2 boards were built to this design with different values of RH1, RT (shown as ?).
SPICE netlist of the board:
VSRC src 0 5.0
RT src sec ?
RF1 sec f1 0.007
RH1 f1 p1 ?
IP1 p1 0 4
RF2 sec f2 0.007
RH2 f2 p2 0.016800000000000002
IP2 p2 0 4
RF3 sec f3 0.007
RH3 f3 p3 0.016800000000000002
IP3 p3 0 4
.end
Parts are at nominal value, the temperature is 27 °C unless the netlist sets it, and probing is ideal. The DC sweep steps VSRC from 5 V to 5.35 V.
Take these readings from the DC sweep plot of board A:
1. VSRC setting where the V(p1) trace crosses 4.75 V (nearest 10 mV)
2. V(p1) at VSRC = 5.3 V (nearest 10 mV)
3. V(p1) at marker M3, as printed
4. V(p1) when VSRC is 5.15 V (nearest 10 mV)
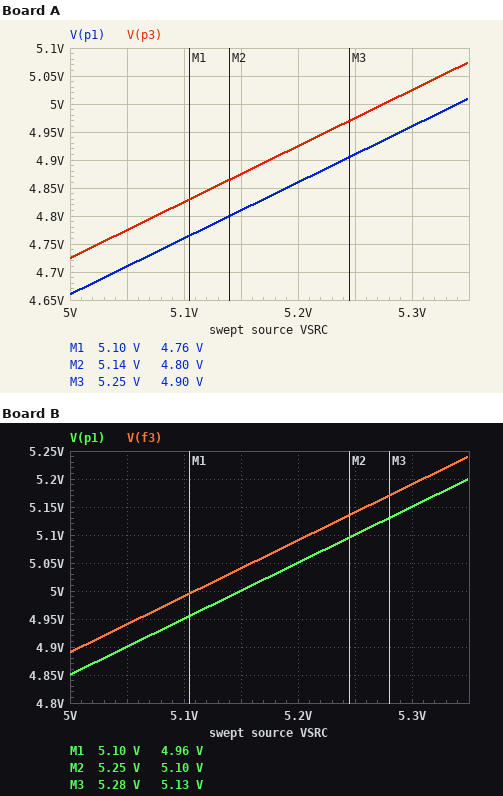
5.09 V
4.96 V
4.90 V
4.81 V
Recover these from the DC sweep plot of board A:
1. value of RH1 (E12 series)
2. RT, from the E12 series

0.033 Ω
0.015 Ω
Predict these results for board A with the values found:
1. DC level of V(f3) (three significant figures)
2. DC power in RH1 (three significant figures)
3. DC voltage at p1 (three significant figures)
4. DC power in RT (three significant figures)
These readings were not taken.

4.79 V
528 mW
4.66 V
2.16 W
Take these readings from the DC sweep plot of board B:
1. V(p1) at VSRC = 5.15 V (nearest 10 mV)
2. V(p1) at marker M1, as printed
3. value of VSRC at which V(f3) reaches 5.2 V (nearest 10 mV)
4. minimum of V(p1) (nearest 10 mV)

5.00 V
4.96 V
5.31 V
4.85 V
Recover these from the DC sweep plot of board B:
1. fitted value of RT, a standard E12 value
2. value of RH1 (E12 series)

6.8 mΩ
0.01 Ω
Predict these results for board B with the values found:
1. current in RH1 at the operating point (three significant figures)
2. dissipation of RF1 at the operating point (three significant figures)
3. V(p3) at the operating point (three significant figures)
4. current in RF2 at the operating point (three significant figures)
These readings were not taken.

4.00 A
112 mW
4.82 V
4.00 A
